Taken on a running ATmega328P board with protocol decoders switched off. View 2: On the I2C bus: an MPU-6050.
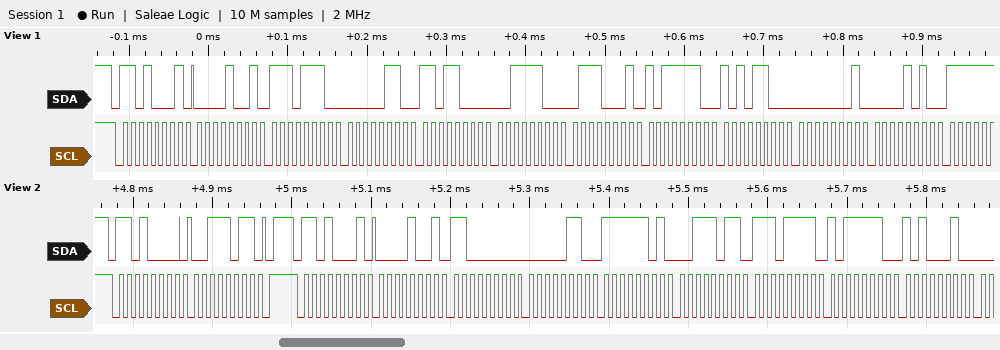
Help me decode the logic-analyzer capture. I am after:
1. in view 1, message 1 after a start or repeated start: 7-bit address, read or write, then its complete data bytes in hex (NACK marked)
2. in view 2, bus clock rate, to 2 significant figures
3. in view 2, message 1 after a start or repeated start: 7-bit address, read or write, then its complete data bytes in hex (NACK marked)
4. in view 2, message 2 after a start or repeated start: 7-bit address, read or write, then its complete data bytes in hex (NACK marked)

0x68 read: 09 EE 06 D8 3C 71 BE AC 01 0A
100 kHz
0x68 write: 3B
0x68 read: 09 C0 06 FD 3B EF BE A2
